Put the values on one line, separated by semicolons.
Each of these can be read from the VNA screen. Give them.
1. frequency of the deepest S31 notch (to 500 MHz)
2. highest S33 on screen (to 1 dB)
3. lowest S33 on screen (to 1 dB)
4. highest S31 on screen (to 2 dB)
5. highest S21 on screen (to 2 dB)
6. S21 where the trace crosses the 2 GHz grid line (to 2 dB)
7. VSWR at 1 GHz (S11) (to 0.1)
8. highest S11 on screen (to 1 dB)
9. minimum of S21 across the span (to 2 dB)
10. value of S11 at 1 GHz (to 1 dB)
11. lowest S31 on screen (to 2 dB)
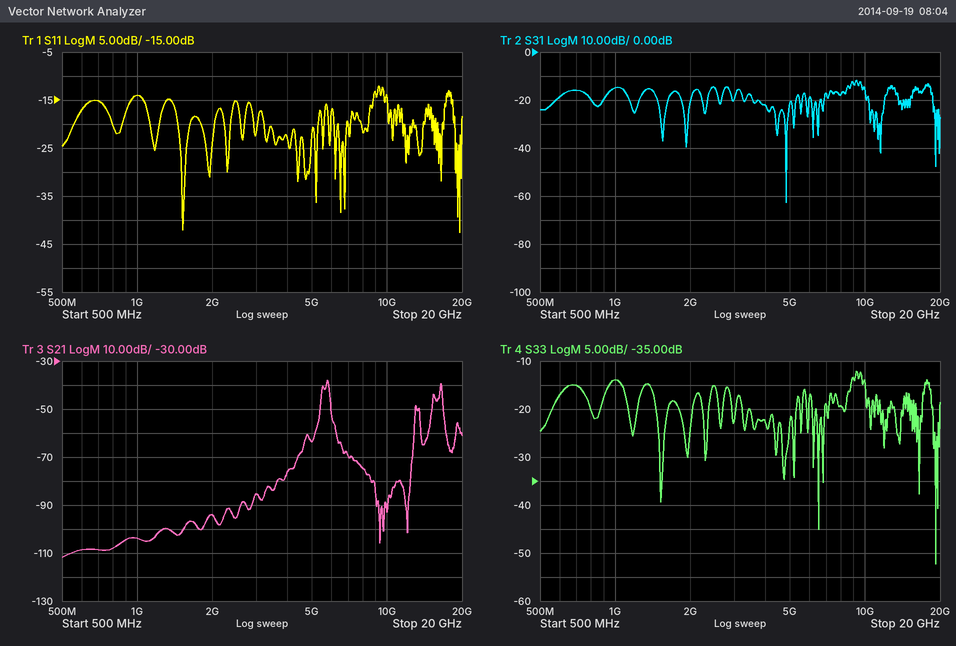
5.0 GHz; -12 dB; -52 dB; -12 dB; -38 dB; -94 dB; 1.5; -12 dB; -112 dB; -14 dB; -62 dB
